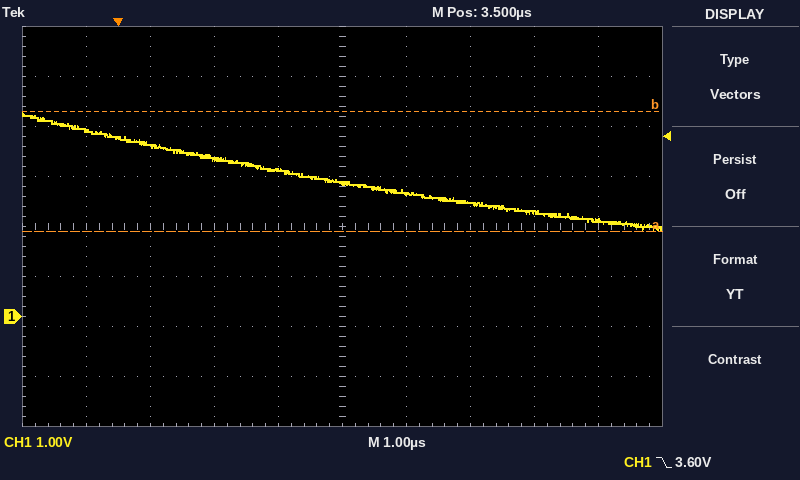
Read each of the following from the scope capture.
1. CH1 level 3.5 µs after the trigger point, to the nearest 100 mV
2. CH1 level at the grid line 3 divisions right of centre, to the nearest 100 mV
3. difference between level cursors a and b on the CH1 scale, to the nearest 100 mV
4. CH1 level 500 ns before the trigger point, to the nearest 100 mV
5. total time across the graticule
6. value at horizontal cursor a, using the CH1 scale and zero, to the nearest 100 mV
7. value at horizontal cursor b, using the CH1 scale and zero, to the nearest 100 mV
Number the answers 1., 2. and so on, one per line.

1. 2.7 V
2. 2.1 V
3. 2.4 V
4. 3.7 V
5. 10 µs
6. 1.7 V
7. 4.1 V
